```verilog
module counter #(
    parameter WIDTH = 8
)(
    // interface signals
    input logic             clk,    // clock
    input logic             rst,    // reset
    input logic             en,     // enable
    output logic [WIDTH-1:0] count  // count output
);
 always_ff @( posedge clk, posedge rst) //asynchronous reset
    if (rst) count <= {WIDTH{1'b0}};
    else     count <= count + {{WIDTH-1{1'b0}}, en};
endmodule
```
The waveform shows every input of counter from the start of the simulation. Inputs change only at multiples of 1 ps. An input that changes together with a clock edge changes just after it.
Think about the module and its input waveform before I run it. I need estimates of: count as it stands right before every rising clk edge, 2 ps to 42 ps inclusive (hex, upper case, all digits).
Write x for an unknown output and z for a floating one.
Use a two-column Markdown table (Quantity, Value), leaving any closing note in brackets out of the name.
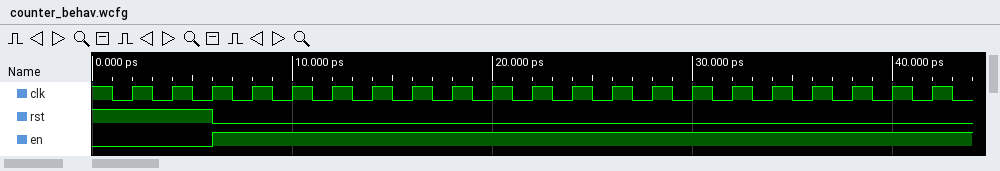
| Quantity | Value |
|---|---|
| count as it stands right before every rising clk edge, 2 ps to 42 ps inclusive | 00, 00, 00, 00, 01, 02, 03, 04, 05, 06, 07, 08, 09, 0A, 0B, 0C, 0D, 0E, 0F, 10, 11 |
